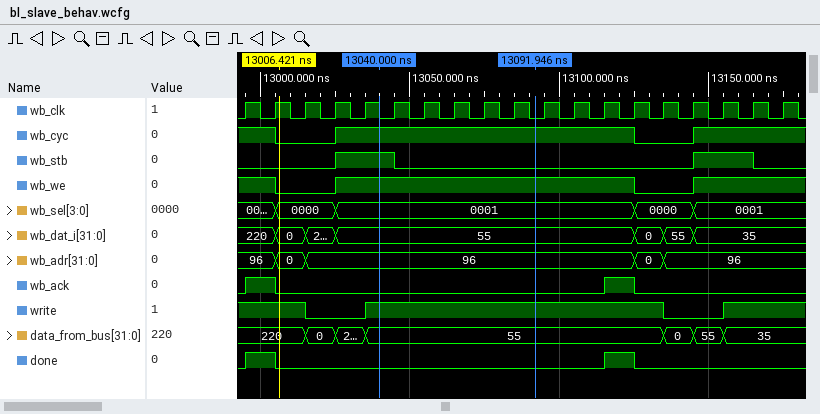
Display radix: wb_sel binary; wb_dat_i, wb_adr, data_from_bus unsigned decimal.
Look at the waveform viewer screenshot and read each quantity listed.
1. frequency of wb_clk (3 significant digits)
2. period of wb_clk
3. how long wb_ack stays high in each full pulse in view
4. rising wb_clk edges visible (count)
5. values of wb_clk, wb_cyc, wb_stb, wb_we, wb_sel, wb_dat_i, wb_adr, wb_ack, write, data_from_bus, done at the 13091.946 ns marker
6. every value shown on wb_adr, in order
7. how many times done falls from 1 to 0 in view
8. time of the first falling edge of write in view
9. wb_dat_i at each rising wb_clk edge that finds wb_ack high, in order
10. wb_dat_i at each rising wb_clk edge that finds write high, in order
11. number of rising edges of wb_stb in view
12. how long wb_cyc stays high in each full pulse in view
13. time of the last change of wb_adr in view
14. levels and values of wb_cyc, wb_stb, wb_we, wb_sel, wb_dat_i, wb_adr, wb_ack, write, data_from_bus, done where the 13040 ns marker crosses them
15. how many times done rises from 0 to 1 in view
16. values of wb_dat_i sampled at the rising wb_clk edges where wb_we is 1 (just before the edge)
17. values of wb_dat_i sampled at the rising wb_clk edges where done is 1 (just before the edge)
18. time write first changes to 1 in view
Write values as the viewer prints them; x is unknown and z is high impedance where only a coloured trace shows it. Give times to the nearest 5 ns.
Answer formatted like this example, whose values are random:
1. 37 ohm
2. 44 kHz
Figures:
1. 100 MHz
2. 10 ns
3. 10 ns, 10 ns
4. 19
5. wb_clk=0, wb_cyc=1, wb_stb=0, wb_we=1, wb_sel=0001, wb_dat_i=55, wb_adr=96, wb_ack=0, write=1, data_from_bus=55, done=0
6. 96, 0, 96, 0, 96
7. 2
8. 13015 ns
9. 220, 55
10. 220, 220, 0, 55, 55, 55, 55, 55, 55, 55, 55, 55, 0, 35, 35
11. 2
12. 100 ns
13. 13135 ns
14. wb_cyc=1, wb_stb=1, wb_we=1, wb_sel=0001, wb_dat_i=55, wb_adr=96, wb_ack=0, write=1, data_from_bus=55, done=0
15. 2
16. 220, 220, 55, 55, 55, 55, 55, 55, 55, 55, 55, 55, 35, 35, 35
17. 220, 55
18. 13035 ns
